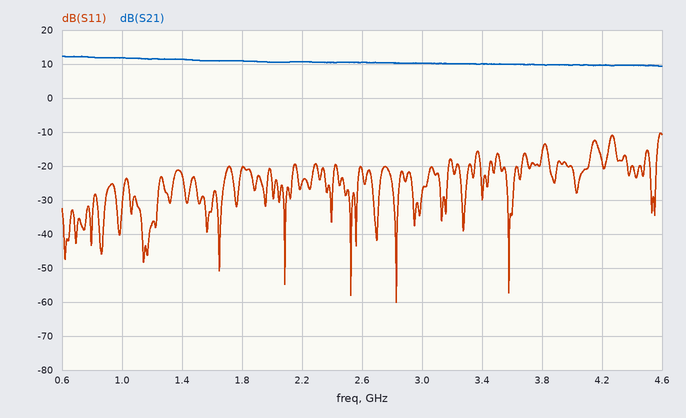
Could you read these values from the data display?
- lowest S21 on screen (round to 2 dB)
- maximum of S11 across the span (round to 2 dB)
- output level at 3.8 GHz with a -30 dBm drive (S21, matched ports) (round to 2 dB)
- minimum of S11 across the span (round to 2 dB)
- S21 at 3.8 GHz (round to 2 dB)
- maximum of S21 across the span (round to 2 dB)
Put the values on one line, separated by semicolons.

10 dB; -10 dB; -20 dBm; -60 dB; 10 dB; 12 dB
